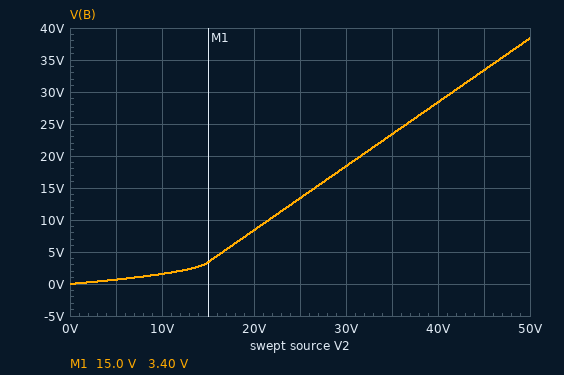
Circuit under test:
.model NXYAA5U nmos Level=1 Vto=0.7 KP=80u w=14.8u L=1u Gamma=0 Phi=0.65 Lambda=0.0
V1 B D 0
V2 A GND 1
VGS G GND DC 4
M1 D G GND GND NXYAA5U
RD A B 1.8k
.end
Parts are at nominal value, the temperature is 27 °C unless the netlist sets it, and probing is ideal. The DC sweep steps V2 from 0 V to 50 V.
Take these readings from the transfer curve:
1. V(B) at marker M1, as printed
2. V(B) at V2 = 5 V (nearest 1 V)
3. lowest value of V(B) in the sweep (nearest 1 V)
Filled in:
3.40 V
1 V
0 V
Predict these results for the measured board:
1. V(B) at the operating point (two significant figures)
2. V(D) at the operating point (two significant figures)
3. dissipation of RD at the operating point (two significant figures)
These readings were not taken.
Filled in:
130 mV
130 mV
420 µW
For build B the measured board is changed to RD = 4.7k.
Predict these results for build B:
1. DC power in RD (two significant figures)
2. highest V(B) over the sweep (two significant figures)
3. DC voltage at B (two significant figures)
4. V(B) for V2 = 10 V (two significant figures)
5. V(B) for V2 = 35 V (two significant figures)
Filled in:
190 µW
20 V
52 mV
560 mV
4.7 V
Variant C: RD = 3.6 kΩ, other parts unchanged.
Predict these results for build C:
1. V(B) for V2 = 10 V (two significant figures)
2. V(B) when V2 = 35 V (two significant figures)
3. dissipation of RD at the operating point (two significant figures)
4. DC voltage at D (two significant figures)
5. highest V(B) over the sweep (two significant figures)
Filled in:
740 mV
12 V
240 µW
67 mV
27 V
